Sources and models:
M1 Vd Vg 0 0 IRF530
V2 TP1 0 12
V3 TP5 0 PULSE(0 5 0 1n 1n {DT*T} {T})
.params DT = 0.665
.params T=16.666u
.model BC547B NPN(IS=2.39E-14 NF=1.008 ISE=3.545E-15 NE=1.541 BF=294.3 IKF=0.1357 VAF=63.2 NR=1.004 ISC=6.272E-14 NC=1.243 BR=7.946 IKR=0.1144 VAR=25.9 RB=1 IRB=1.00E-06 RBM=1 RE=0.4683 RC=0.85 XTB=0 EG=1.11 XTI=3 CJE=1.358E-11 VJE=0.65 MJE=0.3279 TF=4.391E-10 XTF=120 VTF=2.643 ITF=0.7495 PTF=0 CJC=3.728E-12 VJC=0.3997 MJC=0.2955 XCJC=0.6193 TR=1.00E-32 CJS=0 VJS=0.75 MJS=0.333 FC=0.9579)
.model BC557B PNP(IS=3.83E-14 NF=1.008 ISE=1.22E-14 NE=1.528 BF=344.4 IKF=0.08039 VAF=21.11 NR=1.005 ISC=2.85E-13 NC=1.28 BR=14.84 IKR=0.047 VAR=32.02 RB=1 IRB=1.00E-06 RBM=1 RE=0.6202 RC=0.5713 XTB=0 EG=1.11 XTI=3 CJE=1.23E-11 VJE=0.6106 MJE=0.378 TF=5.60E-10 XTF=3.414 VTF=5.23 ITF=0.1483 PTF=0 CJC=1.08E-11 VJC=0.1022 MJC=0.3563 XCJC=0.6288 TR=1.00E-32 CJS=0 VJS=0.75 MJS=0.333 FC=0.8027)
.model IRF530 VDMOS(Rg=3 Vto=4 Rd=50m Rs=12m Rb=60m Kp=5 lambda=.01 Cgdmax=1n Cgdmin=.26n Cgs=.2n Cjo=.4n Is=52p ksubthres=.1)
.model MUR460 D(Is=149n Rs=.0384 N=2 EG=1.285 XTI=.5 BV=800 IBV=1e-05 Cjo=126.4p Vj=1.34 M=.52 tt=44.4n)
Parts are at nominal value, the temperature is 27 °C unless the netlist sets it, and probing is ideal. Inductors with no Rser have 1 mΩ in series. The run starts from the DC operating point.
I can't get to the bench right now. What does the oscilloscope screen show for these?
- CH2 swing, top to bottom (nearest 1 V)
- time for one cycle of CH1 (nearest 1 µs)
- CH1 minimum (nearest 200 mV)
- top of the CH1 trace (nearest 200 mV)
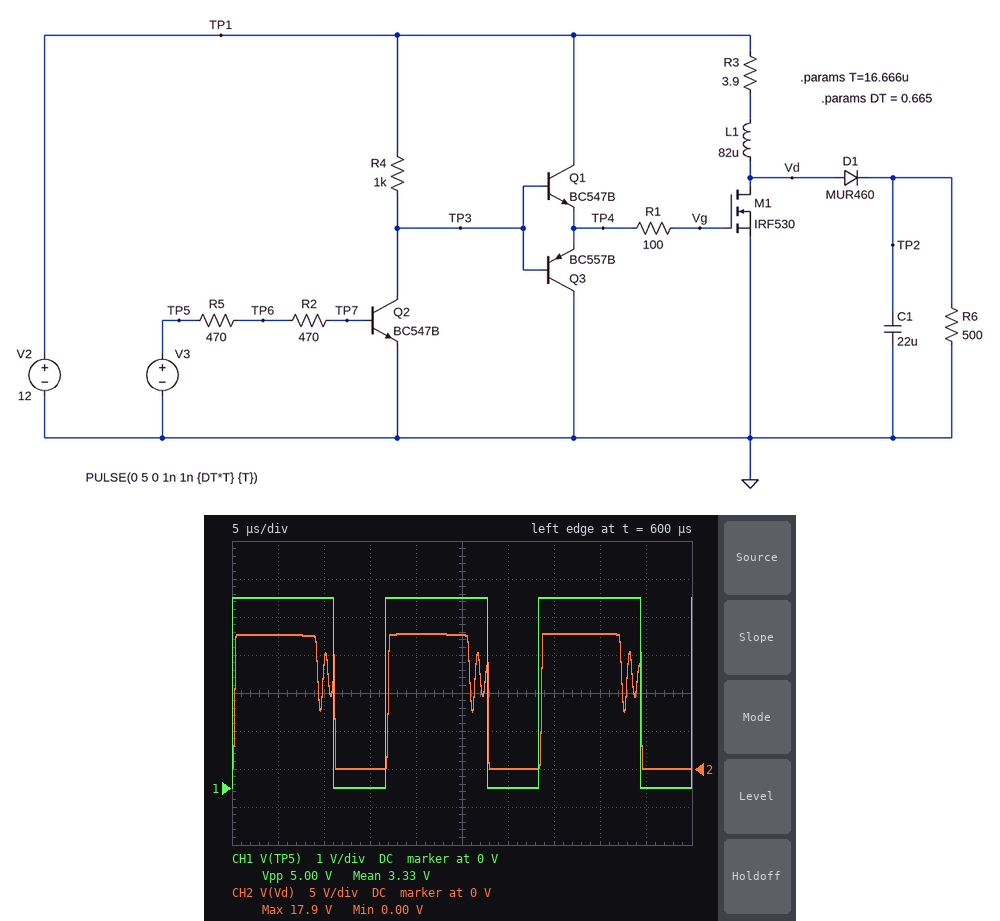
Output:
18 V
17 µs
0 V
5.0 V
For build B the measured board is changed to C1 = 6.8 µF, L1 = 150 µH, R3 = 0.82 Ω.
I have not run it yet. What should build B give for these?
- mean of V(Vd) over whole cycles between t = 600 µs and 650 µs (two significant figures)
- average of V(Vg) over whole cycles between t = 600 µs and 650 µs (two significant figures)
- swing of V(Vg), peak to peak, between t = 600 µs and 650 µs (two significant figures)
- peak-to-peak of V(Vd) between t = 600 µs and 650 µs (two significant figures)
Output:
12 V
3.9 V
17 V
57 V
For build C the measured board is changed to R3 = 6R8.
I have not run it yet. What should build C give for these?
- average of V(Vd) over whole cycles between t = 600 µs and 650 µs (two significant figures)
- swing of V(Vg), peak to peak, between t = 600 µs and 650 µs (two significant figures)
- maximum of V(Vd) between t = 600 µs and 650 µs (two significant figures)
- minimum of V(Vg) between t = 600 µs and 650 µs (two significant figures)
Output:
9.8 V
11 V
15 V
420 mV
